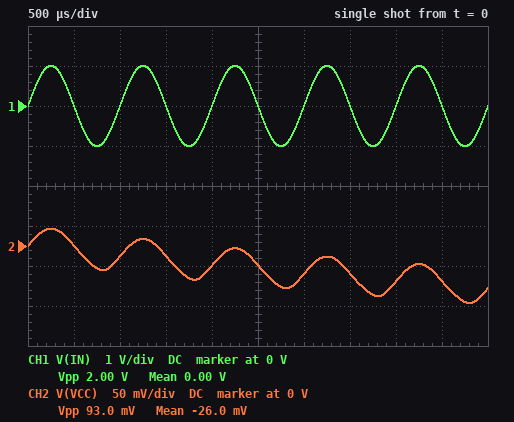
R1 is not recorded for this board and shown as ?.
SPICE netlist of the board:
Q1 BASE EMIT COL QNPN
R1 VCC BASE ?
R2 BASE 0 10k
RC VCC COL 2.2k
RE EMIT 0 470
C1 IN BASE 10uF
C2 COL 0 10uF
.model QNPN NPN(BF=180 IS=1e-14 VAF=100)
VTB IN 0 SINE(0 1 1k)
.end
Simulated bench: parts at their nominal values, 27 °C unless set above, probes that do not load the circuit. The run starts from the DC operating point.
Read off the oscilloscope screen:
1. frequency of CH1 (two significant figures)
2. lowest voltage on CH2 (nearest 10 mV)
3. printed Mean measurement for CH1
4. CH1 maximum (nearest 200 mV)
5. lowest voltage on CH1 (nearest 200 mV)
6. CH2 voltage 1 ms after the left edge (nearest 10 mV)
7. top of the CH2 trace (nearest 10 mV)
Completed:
1.0 kHz
-70 mV
0.00 V
1.0 V
-1.0 V
-10 mV
20 mV
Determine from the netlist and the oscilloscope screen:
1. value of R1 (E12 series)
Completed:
100 kΩ
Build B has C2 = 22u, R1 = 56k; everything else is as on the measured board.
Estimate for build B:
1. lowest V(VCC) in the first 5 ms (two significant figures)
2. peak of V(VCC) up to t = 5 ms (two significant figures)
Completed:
-57 mV
38 mV
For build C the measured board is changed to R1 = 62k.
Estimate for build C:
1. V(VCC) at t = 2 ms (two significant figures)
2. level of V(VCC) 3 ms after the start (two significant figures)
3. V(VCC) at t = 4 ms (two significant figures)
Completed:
-23 mV
-33 mV
-42 mV
